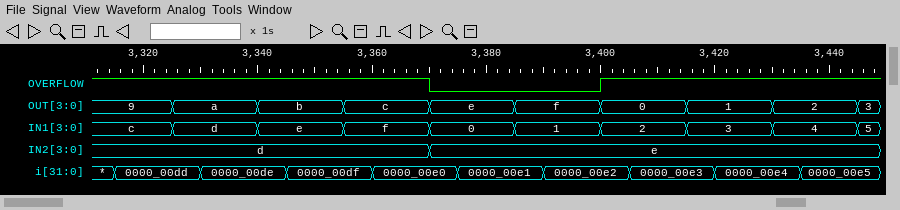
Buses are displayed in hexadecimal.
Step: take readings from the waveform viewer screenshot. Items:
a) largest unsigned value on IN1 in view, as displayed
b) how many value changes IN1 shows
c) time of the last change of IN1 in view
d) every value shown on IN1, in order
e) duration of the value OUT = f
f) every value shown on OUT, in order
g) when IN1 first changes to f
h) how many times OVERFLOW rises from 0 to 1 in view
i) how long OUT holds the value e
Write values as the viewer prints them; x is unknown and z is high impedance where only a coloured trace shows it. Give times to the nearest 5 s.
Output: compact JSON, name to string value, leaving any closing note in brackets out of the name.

{"largest unsigned value on IN1 in view, as displayed": "f", "how many value changes IN1 shows": "9", "time of the last change of IN1 in view": "3445 s", "every value shown on IN1, in order": "c, d, e, f, 0, 1, 2, 3, 4, 5", "duration of the value OUT = f": "15 s", "every value shown on OUT, in order": "9, a, b, c, e, f, 0, 1, 2, 3", "when IN1 first changes to f": "3355 s", "how many times OVERFLOW rises from 0 to 1 in view": "1", "how long OUT holds the value e": "15 s"}
